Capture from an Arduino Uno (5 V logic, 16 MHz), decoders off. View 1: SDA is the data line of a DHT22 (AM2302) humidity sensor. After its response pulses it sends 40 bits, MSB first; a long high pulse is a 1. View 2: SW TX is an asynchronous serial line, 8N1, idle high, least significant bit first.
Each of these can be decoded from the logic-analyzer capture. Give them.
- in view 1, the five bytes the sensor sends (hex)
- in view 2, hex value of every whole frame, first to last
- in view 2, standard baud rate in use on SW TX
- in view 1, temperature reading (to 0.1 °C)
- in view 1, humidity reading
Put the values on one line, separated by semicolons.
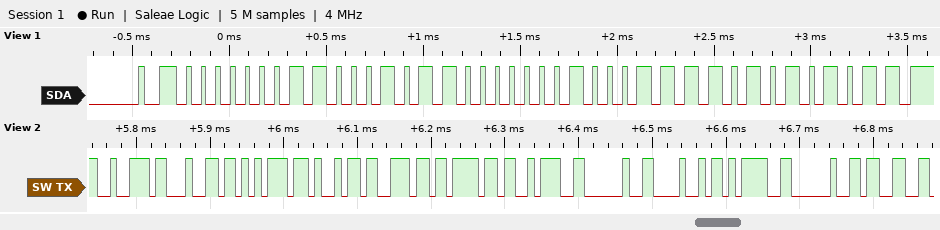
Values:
01 8B 01 1E AB; 0x72 0x64 0x75 0x69 0x6E 0x6F 0x3A 0x20 0x48 0x3D 0x20 0x33; 115200 baud; 28.6 °C; 39.5 %
